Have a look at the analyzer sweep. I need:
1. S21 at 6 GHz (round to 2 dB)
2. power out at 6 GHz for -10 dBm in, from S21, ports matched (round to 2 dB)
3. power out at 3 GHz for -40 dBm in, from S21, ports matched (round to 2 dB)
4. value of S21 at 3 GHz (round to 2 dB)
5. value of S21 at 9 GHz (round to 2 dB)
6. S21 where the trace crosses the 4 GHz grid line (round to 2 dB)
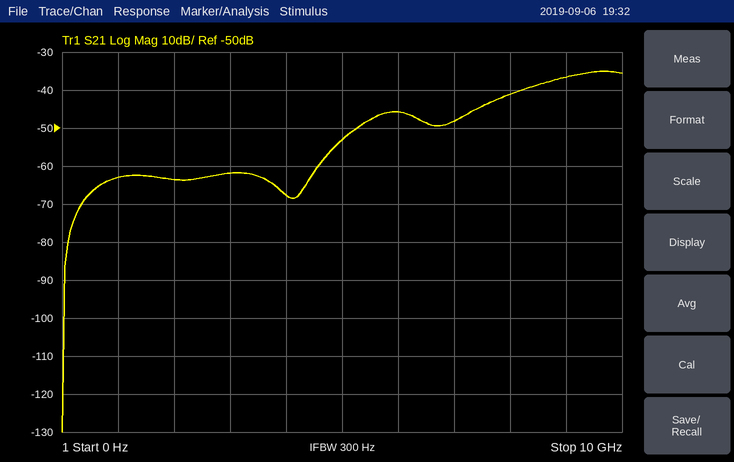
-46 dB
-56 dBm
-102 dBm
-62 dB
-36 dB
-68 dB
